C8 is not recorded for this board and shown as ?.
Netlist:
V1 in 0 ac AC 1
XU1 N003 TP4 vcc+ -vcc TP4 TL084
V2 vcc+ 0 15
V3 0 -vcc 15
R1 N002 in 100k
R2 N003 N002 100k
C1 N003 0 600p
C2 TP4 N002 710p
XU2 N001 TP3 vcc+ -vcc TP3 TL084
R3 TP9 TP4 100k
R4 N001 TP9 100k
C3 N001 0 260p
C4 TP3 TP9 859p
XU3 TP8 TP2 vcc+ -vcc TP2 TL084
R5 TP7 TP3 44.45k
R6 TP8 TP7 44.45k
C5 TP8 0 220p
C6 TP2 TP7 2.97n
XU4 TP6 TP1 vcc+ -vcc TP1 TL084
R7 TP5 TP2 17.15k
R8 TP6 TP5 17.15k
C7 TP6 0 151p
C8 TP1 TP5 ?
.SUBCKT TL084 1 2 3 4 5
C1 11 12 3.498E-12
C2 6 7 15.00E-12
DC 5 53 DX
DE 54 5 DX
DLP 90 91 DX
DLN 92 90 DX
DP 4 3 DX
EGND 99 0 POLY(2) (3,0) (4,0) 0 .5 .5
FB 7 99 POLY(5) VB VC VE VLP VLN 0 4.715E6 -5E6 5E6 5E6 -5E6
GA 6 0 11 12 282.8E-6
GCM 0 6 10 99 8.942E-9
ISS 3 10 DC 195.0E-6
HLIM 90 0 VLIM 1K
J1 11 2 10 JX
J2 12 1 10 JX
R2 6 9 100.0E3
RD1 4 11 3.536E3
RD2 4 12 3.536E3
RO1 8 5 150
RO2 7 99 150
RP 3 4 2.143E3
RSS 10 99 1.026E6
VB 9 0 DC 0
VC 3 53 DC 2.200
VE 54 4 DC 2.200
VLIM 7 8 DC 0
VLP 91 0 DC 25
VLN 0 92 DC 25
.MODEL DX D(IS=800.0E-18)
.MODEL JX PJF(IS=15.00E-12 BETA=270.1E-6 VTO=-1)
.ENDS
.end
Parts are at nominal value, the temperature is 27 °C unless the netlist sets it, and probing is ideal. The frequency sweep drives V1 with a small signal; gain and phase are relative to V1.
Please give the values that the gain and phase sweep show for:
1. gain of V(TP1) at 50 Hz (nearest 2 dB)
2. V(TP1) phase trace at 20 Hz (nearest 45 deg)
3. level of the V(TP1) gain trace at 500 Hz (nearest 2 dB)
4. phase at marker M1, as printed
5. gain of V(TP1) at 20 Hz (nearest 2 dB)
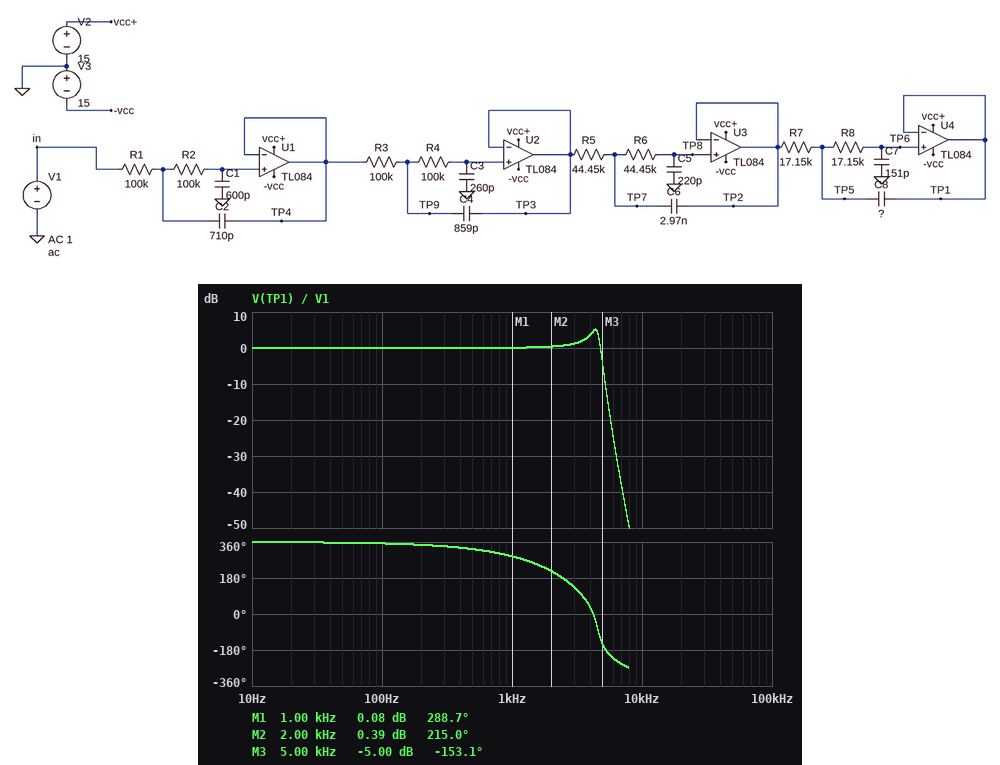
0 dB
360 deg
0 dB
288.7 deg
0 dB
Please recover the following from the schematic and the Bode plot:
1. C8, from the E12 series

27 nF
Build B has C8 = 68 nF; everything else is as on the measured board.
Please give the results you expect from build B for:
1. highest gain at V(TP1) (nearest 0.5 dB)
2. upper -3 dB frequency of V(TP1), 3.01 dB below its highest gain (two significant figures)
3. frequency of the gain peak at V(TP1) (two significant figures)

17.5 dB
3.0 kHz
2.9 kHz
